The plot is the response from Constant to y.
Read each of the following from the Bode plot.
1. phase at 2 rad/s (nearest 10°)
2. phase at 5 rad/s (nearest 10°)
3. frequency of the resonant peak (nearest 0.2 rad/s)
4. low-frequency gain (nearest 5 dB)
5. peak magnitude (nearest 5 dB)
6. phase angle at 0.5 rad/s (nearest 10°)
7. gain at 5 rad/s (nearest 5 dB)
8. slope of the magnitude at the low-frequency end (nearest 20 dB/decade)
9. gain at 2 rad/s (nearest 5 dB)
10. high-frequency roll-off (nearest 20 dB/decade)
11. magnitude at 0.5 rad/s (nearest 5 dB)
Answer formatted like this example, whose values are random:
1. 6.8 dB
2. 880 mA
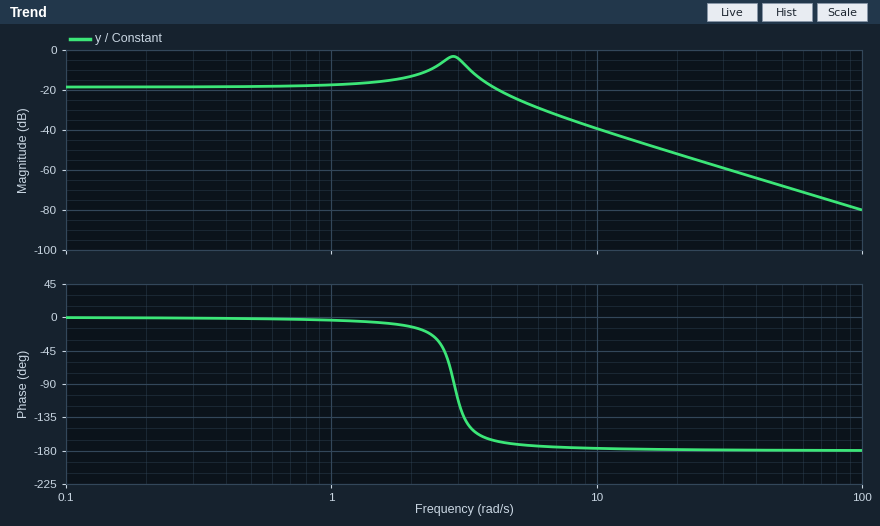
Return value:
1. -10°
2. -170°
3. 2.8 rad/s
4. -20 dB
5. -5 dB
6. 0°
7. -25 dB
8. 0 dB/decade
9. -15 dB
10. -40 dB/decade
11. -20 dB
